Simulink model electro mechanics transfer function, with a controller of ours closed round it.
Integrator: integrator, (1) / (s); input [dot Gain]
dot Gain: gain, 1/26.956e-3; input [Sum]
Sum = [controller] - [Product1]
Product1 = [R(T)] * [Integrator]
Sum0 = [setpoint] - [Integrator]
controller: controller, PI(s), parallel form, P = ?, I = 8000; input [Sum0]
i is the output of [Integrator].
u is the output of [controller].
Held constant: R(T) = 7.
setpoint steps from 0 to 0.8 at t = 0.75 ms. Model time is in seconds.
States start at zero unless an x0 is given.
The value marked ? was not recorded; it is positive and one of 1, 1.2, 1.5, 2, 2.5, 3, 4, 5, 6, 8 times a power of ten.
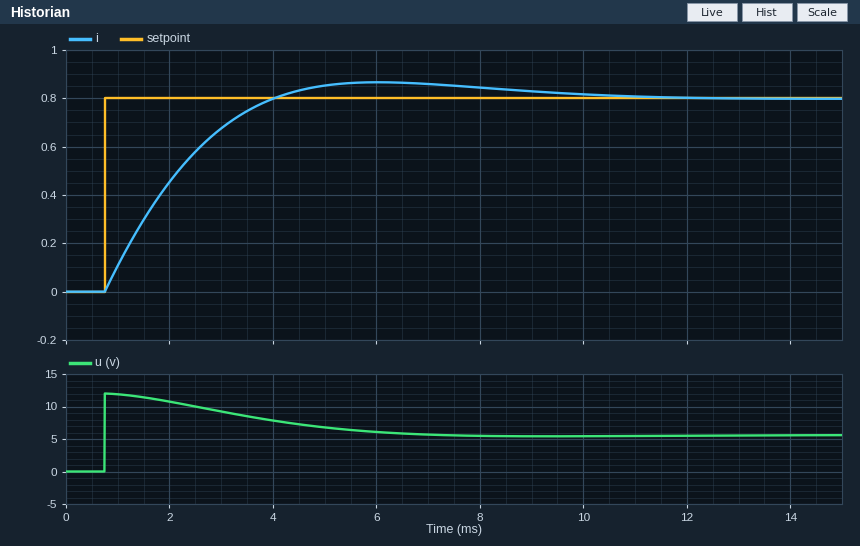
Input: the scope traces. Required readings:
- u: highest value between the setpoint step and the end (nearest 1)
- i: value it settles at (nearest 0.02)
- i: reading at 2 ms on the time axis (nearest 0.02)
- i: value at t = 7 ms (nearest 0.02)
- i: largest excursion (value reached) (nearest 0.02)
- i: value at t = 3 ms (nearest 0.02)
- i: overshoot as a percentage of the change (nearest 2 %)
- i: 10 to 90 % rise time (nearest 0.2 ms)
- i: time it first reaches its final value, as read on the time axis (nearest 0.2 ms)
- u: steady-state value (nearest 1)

12
0.80
0.46
0.86
0.86
0.68
8 %
2.4 ms
4.0 ms
6
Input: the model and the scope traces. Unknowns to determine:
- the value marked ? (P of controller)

15
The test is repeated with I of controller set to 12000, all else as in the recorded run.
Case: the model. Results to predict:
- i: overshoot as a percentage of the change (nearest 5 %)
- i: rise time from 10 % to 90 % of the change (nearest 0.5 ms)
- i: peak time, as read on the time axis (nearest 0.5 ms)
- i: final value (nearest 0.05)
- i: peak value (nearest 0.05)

15 %
2.0 ms
5.0 ms
0.80
0.90
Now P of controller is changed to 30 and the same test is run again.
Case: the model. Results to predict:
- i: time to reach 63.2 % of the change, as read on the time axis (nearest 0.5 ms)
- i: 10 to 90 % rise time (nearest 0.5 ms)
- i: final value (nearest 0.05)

1.5 ms
2.0 ms
0.80
